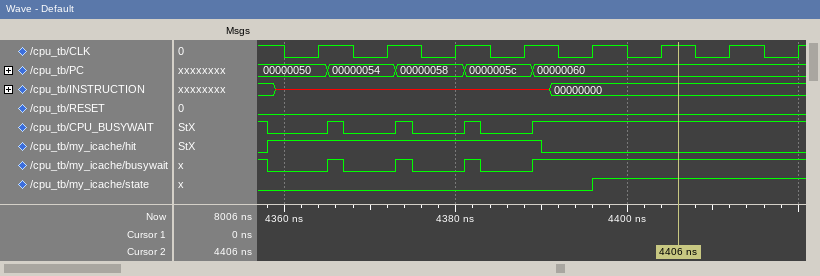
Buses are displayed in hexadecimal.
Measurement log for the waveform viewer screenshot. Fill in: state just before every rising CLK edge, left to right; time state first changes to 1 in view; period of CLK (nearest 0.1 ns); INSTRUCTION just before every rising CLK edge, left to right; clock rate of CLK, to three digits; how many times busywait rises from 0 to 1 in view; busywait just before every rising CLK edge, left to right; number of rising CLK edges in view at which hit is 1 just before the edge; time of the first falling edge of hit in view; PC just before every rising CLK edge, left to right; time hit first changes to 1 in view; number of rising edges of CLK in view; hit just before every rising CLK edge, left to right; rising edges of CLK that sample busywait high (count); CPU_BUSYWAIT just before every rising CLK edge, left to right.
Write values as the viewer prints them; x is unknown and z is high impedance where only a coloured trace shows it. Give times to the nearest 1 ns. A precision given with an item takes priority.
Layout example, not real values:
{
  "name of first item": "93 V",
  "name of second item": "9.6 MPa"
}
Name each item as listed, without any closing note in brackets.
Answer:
{
  "state just before every rising CLK edge, left to right": "0 0 0 0 0 1 1 1",
  "time state first changes to 1 in view": "4396 ns",
  "period of CLK": "8 ns",
  "INSTRUCTION just before every rising CLK edge, left to right": "x, x, x, x, 00000000, 00000000, 00000000, 00000000",
  "clock rate of CLK, to three digits": "125 MHz",
  "how many times busywait rises from 0 to 1 in view": "4",
  "busywait just before every rising CLK edge, left to right": "0 0 0 0 1 1 1 1",
  "number of rising CLK edges in view at which hit is 1 just before the edge": "4",
  "time of the first falling edge of hit in view": "4390 ns",
  "PC just before every rising CLK edge, left to right": "00000050, 00000054, 00000058, 0000005c, 00000060, 00000060, 00000060, 00000060",
  "time hit first changes to 1 in view": "4358 ns",
  "number of rising edges of CLK in view": "8",
  "hit just before every rising CLK edge, left to right": "1 1 1 1 0 0 0 0",
  "rising edges of CLK that sample busywait high": "4",
  "CPU_BUSYWAIT just before every rising CLK edge, left to right": "0 0 0 0 1 1 1 1"
}
